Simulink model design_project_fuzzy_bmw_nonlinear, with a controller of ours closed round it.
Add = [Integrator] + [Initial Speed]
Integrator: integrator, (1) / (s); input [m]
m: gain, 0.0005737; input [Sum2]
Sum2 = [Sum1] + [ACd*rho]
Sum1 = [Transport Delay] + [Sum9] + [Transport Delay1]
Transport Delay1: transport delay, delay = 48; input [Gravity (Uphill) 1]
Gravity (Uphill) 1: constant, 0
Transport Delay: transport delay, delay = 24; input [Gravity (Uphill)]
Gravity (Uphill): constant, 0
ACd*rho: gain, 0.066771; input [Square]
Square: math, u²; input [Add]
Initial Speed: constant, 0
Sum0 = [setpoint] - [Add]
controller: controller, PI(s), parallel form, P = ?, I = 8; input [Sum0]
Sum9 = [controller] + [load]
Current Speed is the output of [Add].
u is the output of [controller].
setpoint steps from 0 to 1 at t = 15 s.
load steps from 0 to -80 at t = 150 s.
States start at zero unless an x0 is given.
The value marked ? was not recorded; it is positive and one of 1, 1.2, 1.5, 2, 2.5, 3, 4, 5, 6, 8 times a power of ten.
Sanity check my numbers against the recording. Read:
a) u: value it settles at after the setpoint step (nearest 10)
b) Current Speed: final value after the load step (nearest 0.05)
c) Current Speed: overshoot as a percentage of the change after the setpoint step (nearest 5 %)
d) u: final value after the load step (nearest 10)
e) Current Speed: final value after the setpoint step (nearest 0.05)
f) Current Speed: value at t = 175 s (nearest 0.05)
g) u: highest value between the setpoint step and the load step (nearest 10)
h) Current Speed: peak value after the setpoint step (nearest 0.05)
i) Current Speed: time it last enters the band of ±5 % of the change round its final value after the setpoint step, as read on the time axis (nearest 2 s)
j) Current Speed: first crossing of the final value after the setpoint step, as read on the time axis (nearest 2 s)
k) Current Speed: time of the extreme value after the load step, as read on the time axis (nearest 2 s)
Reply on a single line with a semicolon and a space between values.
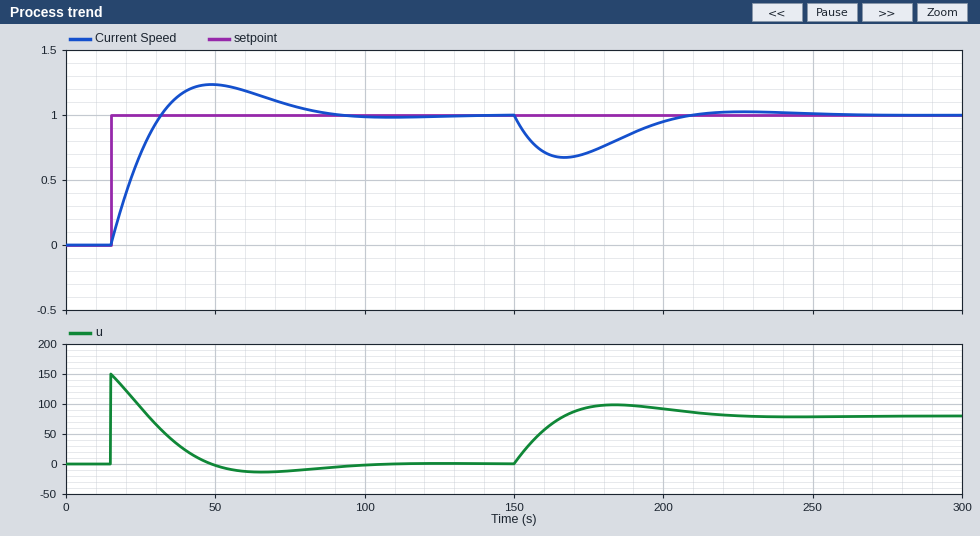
0; 1.00; 25 %; 80; 1.00; 0.70; 150; 1.25; 80 s; 32 s; 166 s
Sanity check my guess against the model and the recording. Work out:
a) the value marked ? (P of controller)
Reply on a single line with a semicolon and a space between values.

150
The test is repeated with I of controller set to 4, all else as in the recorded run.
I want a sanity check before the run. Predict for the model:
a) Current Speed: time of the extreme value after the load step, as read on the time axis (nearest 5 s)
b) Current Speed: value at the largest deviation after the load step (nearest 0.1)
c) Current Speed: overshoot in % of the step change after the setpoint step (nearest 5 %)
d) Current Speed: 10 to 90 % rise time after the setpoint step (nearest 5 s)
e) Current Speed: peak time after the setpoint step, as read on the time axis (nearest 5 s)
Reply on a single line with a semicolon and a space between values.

170 s; 0.6; 15 %; 15 s; 60 s
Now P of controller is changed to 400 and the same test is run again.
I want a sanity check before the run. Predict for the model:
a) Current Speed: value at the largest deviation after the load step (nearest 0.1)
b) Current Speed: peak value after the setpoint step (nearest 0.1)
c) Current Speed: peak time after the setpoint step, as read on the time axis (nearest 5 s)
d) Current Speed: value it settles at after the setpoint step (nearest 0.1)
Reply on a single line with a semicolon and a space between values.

0.8; 1.1; 40 s; 1.0
